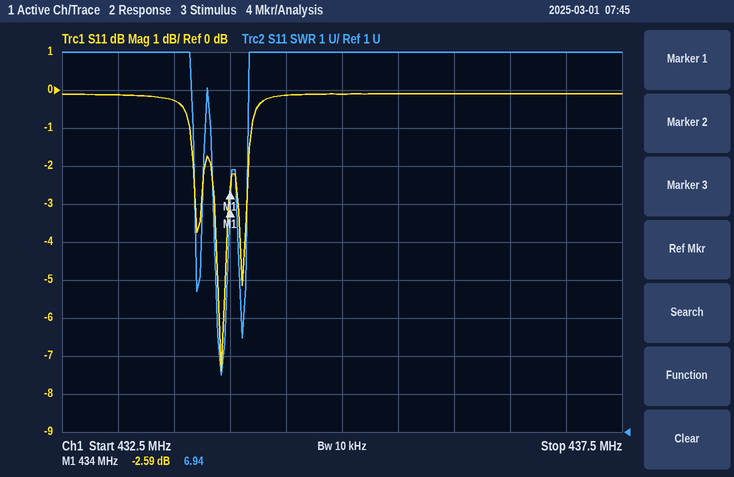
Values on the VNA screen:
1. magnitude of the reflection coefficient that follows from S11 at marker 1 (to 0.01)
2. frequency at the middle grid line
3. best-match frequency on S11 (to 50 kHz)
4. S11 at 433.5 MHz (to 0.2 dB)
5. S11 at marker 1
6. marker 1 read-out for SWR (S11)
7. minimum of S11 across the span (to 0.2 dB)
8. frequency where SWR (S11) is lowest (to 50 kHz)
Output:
0.74
435 MHz
433.90 MHz
-0.2 dB
-2.59 dB
6.94
-7.4 dB
433.90 MHz
